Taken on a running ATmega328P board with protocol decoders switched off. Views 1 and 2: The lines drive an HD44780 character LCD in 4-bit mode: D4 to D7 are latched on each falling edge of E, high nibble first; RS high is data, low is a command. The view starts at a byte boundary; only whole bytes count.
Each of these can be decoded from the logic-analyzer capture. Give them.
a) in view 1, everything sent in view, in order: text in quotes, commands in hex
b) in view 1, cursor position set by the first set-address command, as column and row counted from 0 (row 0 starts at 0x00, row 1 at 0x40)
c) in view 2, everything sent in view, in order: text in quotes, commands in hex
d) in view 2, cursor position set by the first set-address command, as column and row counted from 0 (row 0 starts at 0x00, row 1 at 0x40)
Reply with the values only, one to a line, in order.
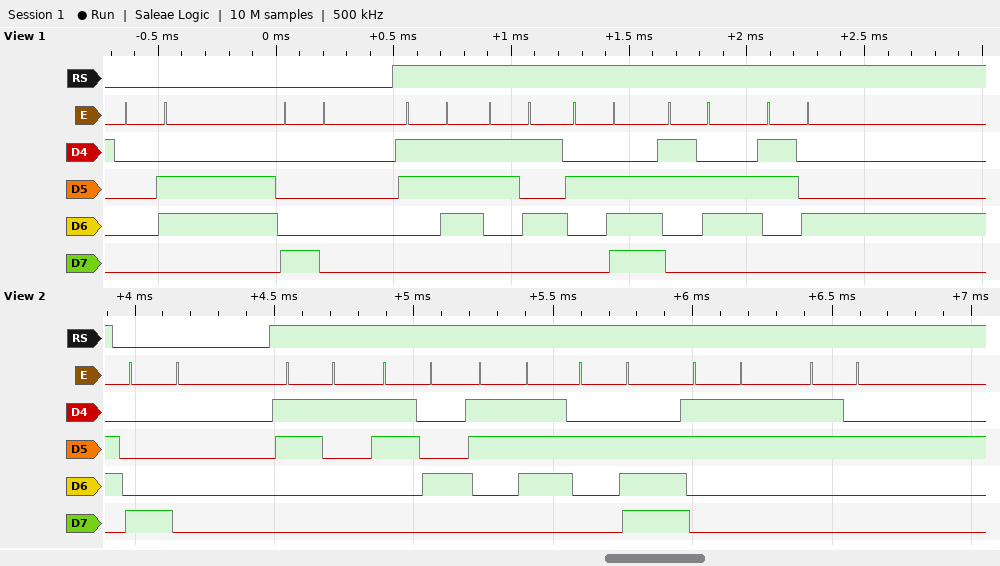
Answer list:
0x06 0x80 "75.64"
column 0, row 0
0x80 "147.32"
column 0, row 0
